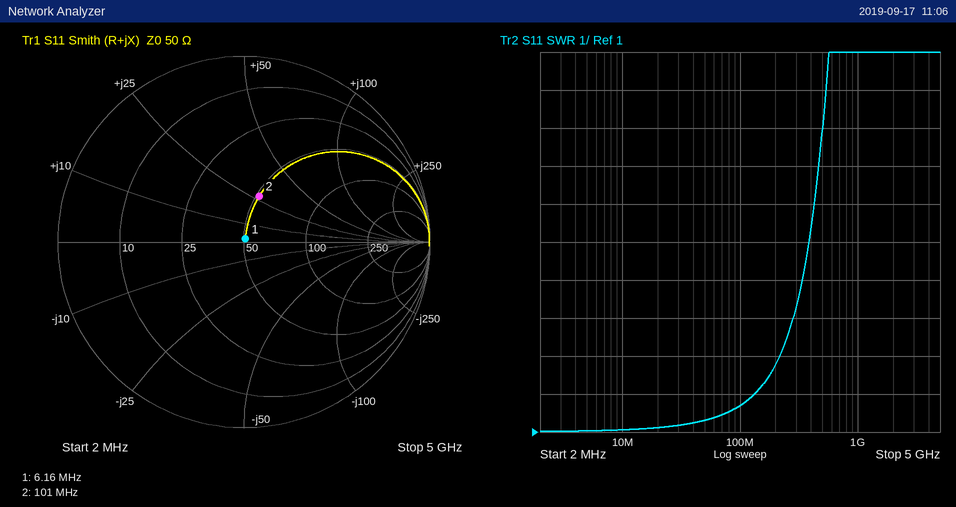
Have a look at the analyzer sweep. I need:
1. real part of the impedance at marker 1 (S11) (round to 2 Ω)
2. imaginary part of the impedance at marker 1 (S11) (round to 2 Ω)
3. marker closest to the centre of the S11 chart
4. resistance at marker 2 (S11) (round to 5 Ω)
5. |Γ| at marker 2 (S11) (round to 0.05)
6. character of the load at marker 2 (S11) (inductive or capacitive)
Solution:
50 Ω
+2 Ω
marker 1
50 Ω
0.25
inductive
